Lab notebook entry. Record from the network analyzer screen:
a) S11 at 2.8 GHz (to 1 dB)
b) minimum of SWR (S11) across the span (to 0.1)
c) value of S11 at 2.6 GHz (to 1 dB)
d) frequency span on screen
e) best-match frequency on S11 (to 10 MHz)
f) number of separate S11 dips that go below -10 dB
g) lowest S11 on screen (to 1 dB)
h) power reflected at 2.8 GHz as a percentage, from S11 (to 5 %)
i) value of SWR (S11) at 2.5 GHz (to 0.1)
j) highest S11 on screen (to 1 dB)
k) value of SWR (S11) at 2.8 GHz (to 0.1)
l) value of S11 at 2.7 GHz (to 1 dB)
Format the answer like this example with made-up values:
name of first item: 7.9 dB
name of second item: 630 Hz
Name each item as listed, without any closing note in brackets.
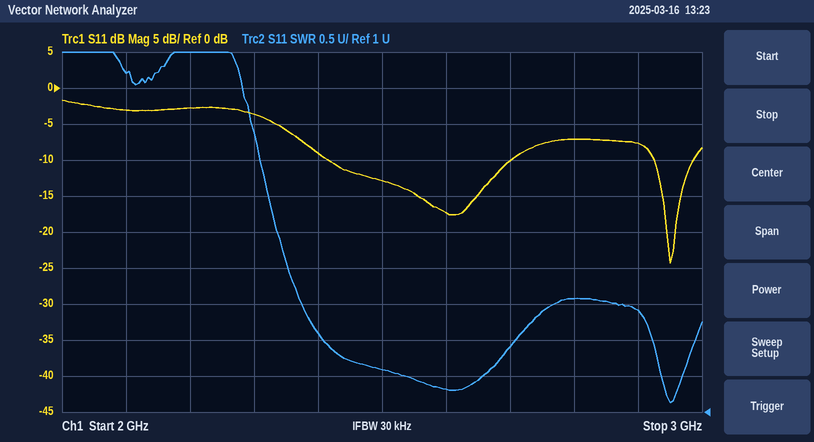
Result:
S11 at 2.8 GHz: -7 dB
minimum of SWR (S11) across the span: 1.1
value of S11 at 2.6 GHz: -17 dB
frequency span on screen: 1 GHz
best-match frequency on S11: 2.95 GHz
number of separate S11 dips that go below -10 dB: 2
lowest S11 on screen: -24 dB
power reflected at 2.8 GHz as a percentage, from S11: 20 %
value of SWR (S11) at 2.5 GHz: 1.6
highest S11 on screen: -2 dB
value of SWR (S11) at 2.8 GHz: 2.6
value of S11 at 2.7 GHz: -10 dB
